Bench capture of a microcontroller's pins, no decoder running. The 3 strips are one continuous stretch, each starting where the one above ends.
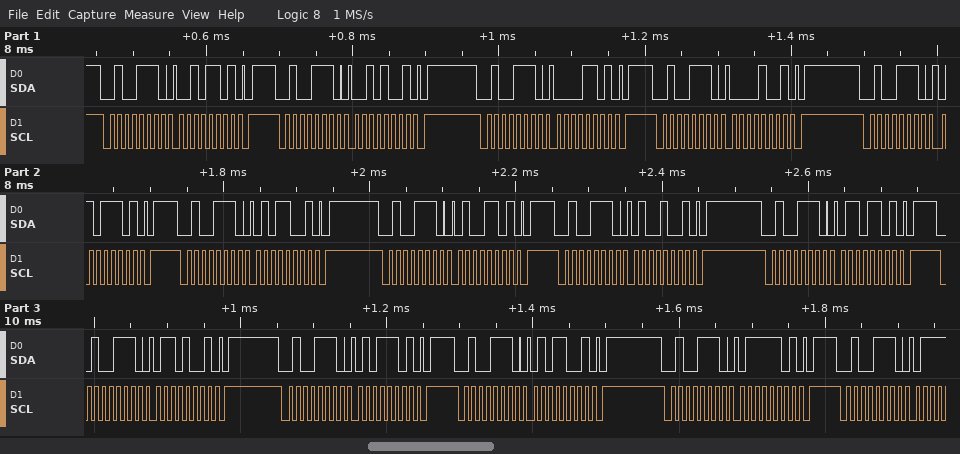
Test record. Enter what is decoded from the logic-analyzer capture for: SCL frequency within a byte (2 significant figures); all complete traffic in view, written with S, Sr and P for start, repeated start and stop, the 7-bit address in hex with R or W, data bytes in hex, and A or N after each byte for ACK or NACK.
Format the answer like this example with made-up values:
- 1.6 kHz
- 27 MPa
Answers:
- 100 kHz
- S 27W A 2D A P S 27W A 29 A P S 27W A 0D A P S 27W A 09 A P S 27W A 5D A P S 27W A 59 A P S 27W A 4D A P S 27W A 49 A P S 27W A 6D A P S 27W A 69 A P S 27W A 5D A P S 27W A 59 A P S 27W A 7D A P S 27W A
